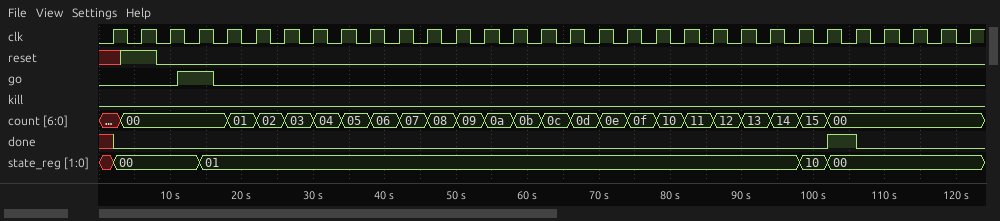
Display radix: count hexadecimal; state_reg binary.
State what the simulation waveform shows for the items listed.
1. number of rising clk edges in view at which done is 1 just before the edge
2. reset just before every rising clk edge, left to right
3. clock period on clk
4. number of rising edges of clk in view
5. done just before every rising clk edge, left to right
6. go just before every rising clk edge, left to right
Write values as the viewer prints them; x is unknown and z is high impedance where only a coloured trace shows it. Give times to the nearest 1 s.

1
x 1 0 0 0 0 0 0 0 0 0 0 0 0 0 0 0 0 0 0 0 0 0 0 0 0 0 0 0 0 0
4 s
31
x 0 0 0 0 0 0 0 0 0 0 0 0 0 0 0 0 0 0 0 0 0 0 0 0 0 1 0 0 0 0
0 0 0 1 0 0 0 0 0 0 0 0 0 0 0 0 0 0 0 0 0 0 0 0 0 0 0 0 0 0 0
